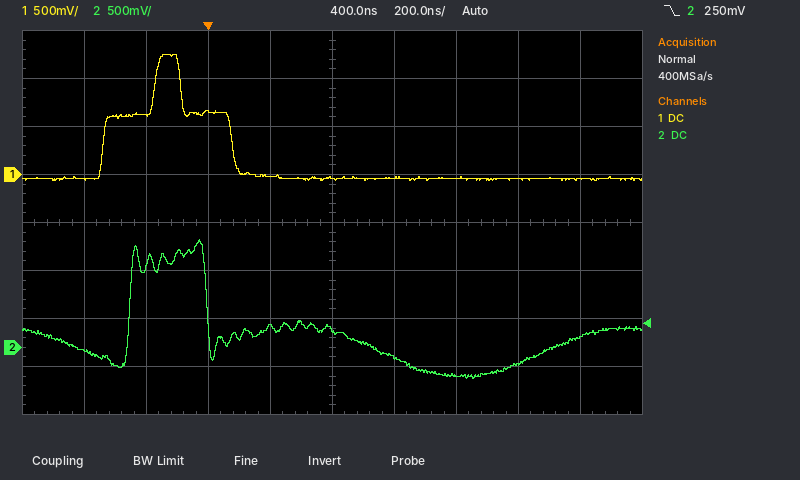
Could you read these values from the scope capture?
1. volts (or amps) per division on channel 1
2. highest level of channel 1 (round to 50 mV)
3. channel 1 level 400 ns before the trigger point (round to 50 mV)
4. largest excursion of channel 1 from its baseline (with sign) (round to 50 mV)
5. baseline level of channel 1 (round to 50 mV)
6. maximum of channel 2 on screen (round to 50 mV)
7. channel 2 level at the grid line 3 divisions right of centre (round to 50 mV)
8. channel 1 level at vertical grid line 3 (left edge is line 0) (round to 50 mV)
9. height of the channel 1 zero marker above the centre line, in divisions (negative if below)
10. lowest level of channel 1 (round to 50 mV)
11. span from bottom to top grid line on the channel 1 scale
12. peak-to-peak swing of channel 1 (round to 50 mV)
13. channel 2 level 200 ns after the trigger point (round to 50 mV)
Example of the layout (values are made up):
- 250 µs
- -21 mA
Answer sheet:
- 500 mV
- 1.25 V
- -50 mV
- +1.30 V
- -50 mV
- 1.10 V
- -150 mV
- 650 mV
- +1.0 div
- -50 mV
- 4 V
- 1.30 V
- 200 mV
